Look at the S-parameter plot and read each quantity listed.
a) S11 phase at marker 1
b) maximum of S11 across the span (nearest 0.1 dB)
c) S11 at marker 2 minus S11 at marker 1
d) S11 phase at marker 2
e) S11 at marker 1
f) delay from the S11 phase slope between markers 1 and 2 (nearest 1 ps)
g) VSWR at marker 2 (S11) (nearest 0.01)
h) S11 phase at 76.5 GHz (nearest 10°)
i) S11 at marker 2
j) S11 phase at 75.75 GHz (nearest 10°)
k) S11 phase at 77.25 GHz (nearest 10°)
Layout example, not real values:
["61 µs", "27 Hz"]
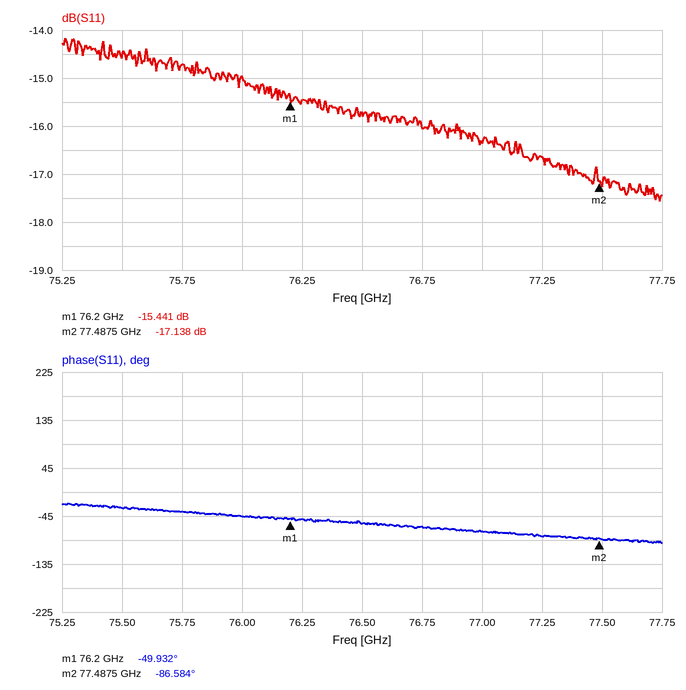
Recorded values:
["-49.932°", "-14.2 dB", "-1.697 dB", "-86.584°", "-15.441 dB", "79 ps", "1.32", "-60°", "-17.138 dB", "-40°", "-80°"]
